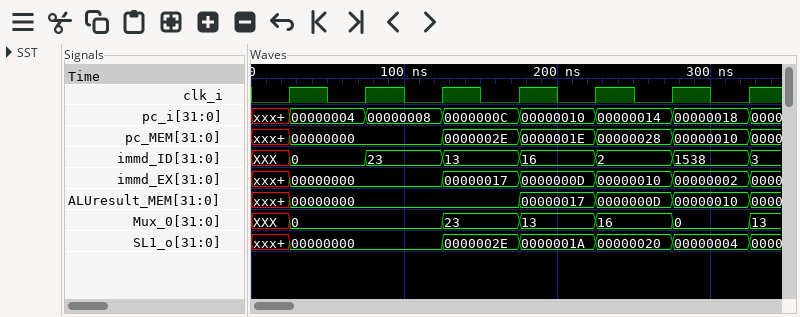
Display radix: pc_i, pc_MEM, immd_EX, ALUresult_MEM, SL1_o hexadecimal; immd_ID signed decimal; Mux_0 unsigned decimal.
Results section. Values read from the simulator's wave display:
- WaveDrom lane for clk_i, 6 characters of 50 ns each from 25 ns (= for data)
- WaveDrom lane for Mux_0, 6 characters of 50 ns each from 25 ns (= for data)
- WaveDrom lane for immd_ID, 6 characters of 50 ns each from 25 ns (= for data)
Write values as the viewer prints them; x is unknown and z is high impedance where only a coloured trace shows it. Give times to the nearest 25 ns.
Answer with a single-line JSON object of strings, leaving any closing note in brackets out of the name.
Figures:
{"WaveDrom lane for clk_i, 6 characters of 50 ns each from 25 ns": "{name: 'clk_i', wave: 'p.....'}", "WaveDrom lane for Mux_0, 6 characters of 50 ns each from 25 ns": "{name: 'Mux_0', wave: '=.====', data: '0 23 13 16 0'}", "WaveDrom lane for immd_ID, 6 characters of 50 ns each from 25 ns": "{name: 'immd_ID', wave: '======', data: '0 23 13 16 2 1538'}"}
